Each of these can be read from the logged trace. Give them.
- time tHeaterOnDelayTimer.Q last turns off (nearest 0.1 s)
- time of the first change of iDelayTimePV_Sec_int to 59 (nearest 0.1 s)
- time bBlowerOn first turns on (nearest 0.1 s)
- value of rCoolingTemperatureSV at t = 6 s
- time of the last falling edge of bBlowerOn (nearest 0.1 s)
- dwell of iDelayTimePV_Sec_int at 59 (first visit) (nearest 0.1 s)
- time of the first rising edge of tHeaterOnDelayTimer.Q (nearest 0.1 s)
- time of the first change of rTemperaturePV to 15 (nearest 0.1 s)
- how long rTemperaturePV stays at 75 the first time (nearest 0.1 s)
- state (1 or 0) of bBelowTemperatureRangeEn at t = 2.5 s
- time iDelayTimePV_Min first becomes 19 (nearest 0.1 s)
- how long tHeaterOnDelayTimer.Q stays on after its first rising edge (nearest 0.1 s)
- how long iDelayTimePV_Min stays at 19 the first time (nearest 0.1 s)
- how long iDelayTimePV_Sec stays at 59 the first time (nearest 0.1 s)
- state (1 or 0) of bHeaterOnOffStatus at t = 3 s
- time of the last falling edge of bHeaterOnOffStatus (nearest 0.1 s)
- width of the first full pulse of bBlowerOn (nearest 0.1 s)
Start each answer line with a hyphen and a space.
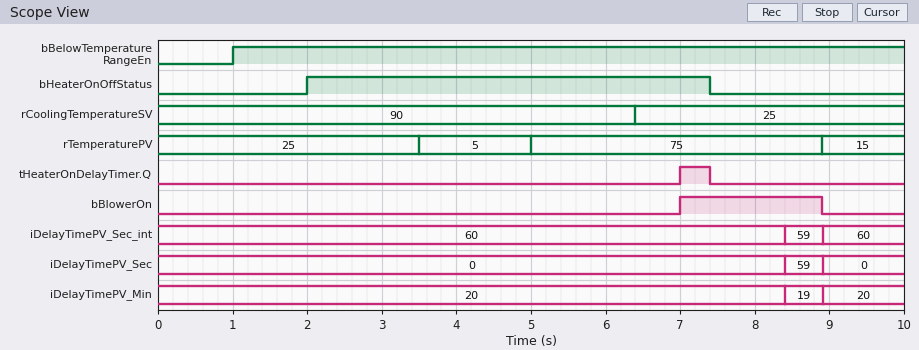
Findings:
- 7.4 s
- 8.4 s
- 7.0 s
- 90
- 8.9 s
- 0.5 s
- 7.0 s
- 8.9 s
- 3.9 s
- 1
- 8.4 s
- 0.4 s
- 0.5 s
- 0.5 s
- 1
- 7.4 s
- 1.9 s
